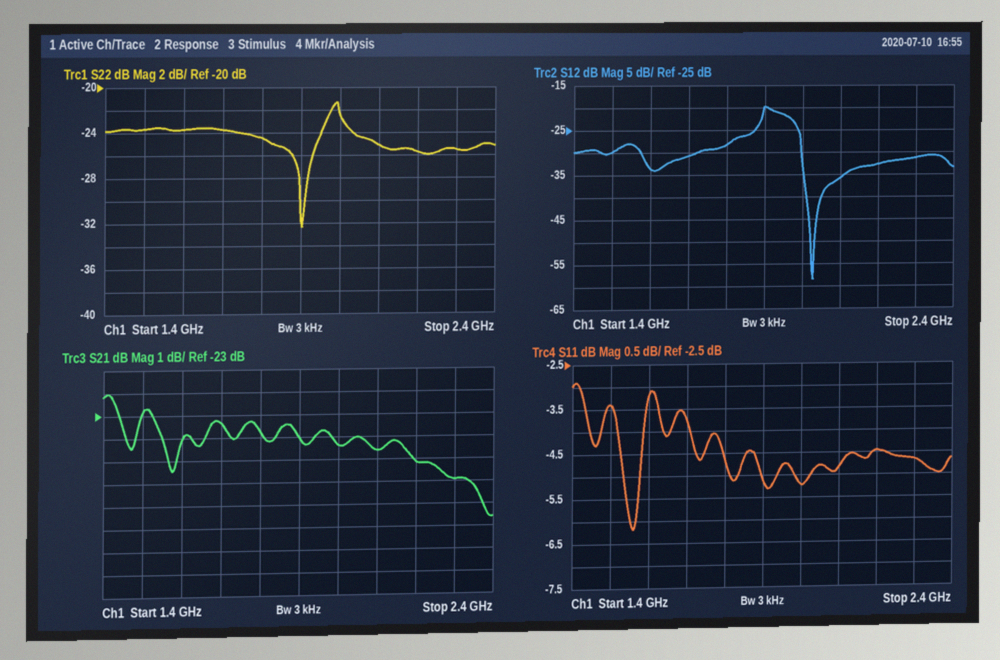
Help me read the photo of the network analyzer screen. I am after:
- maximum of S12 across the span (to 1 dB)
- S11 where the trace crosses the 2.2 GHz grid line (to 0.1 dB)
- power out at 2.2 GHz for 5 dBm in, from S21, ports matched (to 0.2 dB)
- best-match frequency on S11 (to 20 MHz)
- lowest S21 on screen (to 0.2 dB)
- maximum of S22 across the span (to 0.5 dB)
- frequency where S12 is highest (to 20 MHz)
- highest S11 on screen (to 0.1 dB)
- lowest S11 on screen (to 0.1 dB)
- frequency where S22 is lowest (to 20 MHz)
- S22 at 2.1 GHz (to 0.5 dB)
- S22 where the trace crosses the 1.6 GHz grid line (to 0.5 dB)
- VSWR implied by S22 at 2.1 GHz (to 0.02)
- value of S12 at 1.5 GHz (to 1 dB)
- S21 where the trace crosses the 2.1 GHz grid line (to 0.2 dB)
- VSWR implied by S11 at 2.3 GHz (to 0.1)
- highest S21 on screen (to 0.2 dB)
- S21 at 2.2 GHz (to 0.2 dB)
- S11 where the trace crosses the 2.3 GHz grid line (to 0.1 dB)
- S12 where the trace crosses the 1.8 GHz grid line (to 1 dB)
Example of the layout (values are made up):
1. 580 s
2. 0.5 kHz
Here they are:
1. -20 dB
2. -4.5 dB
3. -20.2 dBm
4. 1.56 GHz
5. -27.6 dB
6. -21.5 dB
7. 1.90 GHz
8. -2.9 dB
9. -6.2 dB
10. 1.90 GHz
11. -25.0 dB
12. -23.5 dB
13. 1.12
14. -30 dB
15. -24.6 dB
16. 3.8
17. -22.0 dB
18. -25.2 dB
19. -4.7 dB
20. -28 dB
